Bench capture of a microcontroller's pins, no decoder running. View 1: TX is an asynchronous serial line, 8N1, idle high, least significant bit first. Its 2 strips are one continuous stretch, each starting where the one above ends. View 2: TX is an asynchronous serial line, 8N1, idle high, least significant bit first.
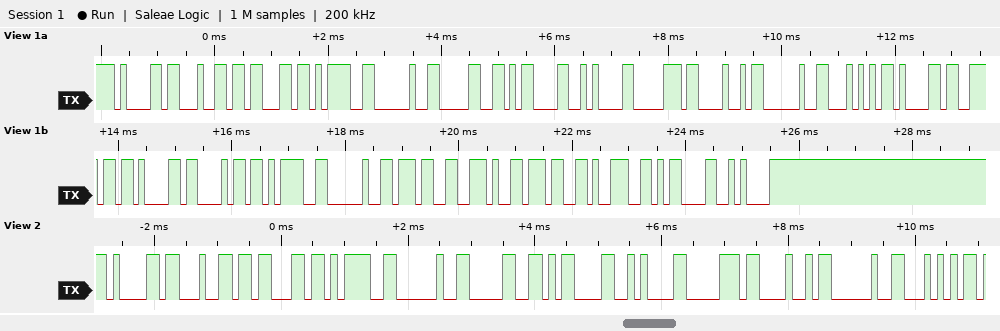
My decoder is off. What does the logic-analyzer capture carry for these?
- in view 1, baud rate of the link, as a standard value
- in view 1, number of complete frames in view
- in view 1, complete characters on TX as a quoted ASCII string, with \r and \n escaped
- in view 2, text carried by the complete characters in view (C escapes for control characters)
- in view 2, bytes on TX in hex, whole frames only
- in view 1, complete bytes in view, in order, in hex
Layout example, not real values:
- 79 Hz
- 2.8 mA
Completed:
- 9600 baud
- 24
- "adc= 0\r\npH Tanah= 7.79\r\n"
- "adc= 0\r\npH T"
- 61 64 63 3D 20 30 0D 0A 70 48 20 54
- 61 64 63 3D 20 30 0D 0A 70 48 20 54 61 6E 61 68 3D 20 37 2E 37 39 0D 0A
